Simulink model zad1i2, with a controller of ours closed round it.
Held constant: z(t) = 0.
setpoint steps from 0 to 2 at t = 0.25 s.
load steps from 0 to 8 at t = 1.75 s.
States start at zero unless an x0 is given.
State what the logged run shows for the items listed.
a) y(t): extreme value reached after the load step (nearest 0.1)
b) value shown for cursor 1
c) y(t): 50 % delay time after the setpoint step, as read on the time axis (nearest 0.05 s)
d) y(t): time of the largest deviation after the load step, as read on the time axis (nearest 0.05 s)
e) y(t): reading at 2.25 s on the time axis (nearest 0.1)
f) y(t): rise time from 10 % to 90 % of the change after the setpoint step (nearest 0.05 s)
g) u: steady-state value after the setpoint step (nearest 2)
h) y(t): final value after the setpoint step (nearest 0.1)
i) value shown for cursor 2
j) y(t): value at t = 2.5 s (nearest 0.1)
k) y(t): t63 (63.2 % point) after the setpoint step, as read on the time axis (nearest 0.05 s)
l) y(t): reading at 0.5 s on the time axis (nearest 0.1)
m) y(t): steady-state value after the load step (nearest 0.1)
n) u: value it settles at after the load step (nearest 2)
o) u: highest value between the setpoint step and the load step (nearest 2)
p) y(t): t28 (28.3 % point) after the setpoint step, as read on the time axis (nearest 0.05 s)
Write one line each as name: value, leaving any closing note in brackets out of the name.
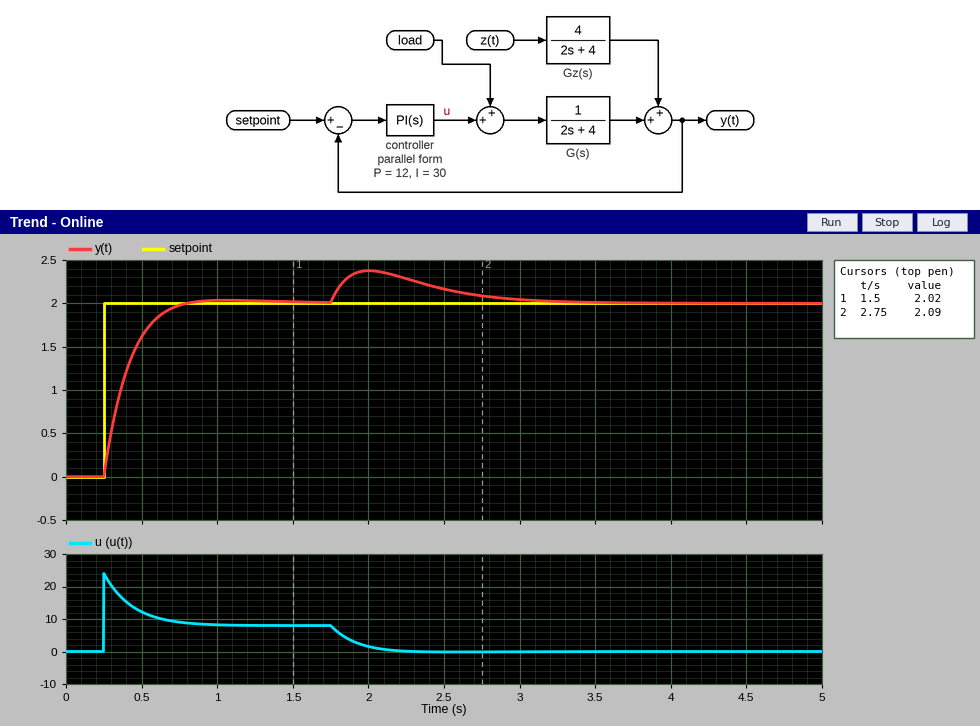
y(t): extreme value reached after the load step: 2.4
value shown for cursor 1: 2.02
y(t): 50 % delay time after the setpoint step, as read on the time axis: 0.35 s
y(t): time of the largest deviation after the load step, as read on the time axis: 2.00 s
y(t): reading at 2.25 s on the time axis: 2.3
y(t): rise time from 10 % to 90 % of the change after the setpoint step: 0.30 s
u: steady-state value after the setpoint step: 8
y(t): final value after the setpoint step: 2.0
value shown for cursor 2: 2.09
y(t): value at t = 2.5 s: 2.2
y(t): t63 (63.2 % point) after the setpoint step, as read on the time axis: 0.40 s
y(t): reading at 0.5 s on the time axis: 1.6
y(t): steady-state value after the load step: 2.0
u: value it settles at after the load step: 0
u: highest value between the setpoint step and the load step: 24
y(t): t28 (28.3 % point) after the setpoint step, as read on the time axis: 0.30 s
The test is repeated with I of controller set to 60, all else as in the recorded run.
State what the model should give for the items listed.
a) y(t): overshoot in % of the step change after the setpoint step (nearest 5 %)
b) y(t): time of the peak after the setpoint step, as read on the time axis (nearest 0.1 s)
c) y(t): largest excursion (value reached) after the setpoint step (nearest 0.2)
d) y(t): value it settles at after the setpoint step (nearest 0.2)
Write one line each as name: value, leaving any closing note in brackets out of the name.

y(t): overshoot in % of the step change after the setpoint step: 10 %
y(t): time of the peak after the setpoint step, as read on the time axis: 0.7 s
y(t): largest excursion (value reached) after the setpoint step: 2.2
y(t): value it settles at after the setpoint step: 2.0
